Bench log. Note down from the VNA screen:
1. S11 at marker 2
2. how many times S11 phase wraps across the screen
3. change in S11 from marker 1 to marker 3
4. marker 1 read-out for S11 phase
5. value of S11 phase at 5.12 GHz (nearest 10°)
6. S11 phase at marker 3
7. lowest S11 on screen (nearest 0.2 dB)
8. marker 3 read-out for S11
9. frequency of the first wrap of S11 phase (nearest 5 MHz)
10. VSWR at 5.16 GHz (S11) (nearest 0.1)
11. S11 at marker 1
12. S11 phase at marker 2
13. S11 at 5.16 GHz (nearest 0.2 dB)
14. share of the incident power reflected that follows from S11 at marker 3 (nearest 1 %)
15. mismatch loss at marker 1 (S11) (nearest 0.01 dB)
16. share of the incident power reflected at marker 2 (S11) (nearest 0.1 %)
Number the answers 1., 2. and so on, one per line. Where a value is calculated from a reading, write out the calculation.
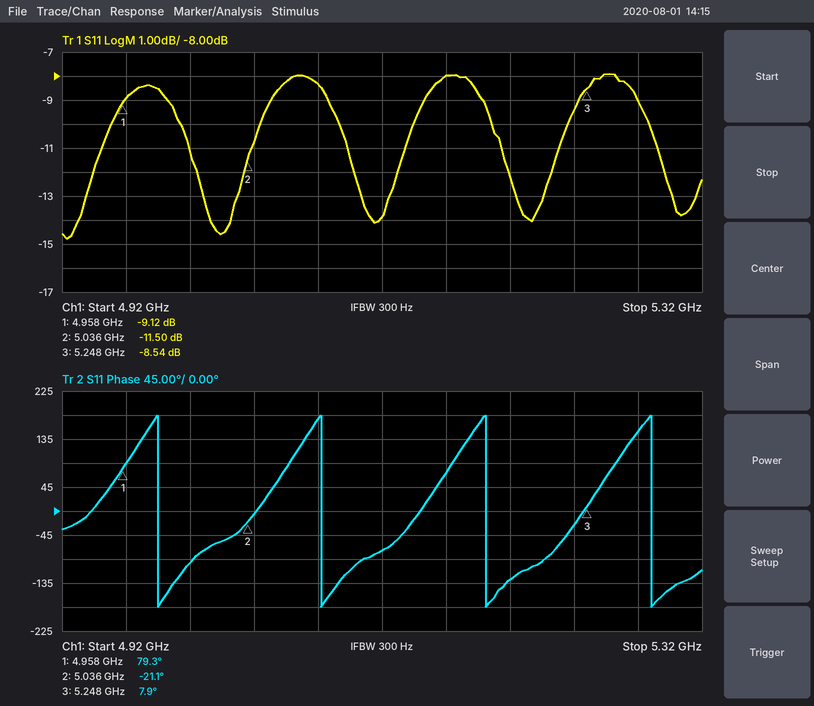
1. -11.50 dB
2. 4
3. -8.54 − (-9.12) = 0.58 dB
4. 79.3°
5. -70°
6. 7.9°
7. -14.8 dB
8. -8.54 dB
9. 4.980 GHz
10. |Γ| = 10^(-8/20) = 0.3981; VSWR = (1 + 0.3981)/(1 − 0.3981) ≈ 2.3
11. -9.12 dB
12. -21.1°
13. -8.0 dB
14. 10^(-8.54/10) ≈ 14 %
15. −10 log10(1 − 10^(-9.12/10)) ≈ 0.57 dB
16. 10^(-11.5/10) ≈ 7.1 %
